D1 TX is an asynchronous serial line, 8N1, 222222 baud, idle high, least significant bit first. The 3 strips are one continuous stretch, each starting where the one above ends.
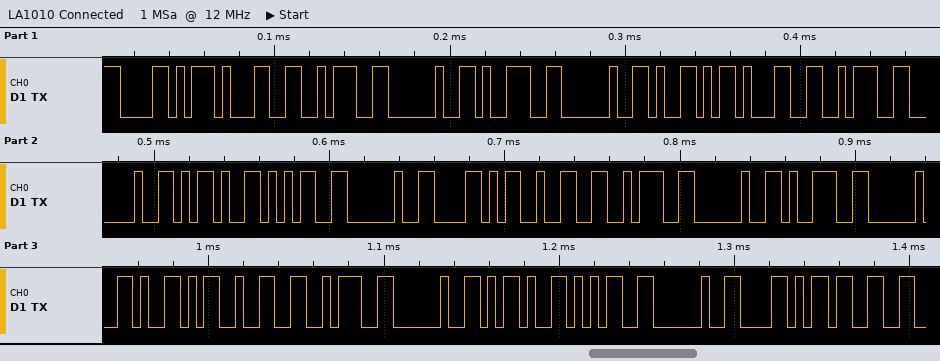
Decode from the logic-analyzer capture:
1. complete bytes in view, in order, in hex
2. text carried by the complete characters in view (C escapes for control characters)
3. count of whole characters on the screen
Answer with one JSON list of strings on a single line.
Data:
["58 31 3A 20 39 20 59 31 3A 20 2D 35 20 58 32 3A 20 39 20 59 32 3A 20 2D 35 20 58 33", "\"X1: 9 Y1: -5 X2: 9 Y2: -5 X3\"", "28"]
